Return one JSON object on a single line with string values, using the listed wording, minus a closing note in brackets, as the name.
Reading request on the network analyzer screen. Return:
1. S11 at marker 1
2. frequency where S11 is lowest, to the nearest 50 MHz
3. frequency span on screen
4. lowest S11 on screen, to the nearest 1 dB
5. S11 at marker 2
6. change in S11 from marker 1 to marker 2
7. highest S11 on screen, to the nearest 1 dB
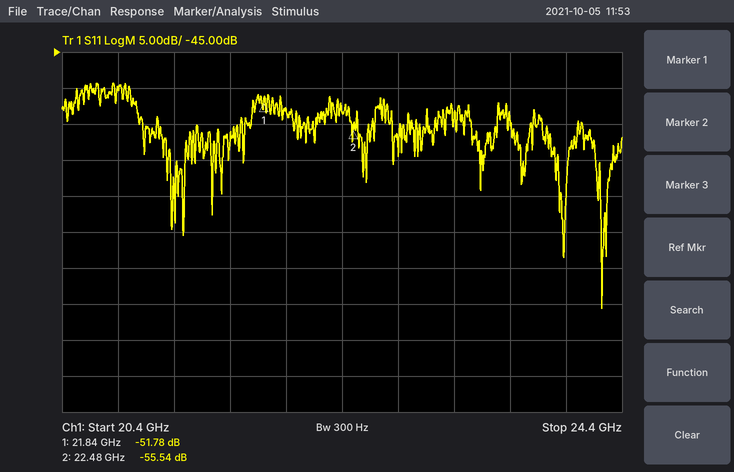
{"S11 at marker 1": "-51.78 dB", "frequency where S11 is lowest, to the nearest 50 MHz": "24.25 GHz", "frequency span on screen": "4 GHz", "lowest S11 on screen, to the nearest 1 dB": "-81 dB", "S11 at marker 2": "-55.54 dB", "change in S11 from marker 1 to marker 2": "-3.76 dB", "highest S11 on screen, to the nearest 1 dB": "-49 dB"}
